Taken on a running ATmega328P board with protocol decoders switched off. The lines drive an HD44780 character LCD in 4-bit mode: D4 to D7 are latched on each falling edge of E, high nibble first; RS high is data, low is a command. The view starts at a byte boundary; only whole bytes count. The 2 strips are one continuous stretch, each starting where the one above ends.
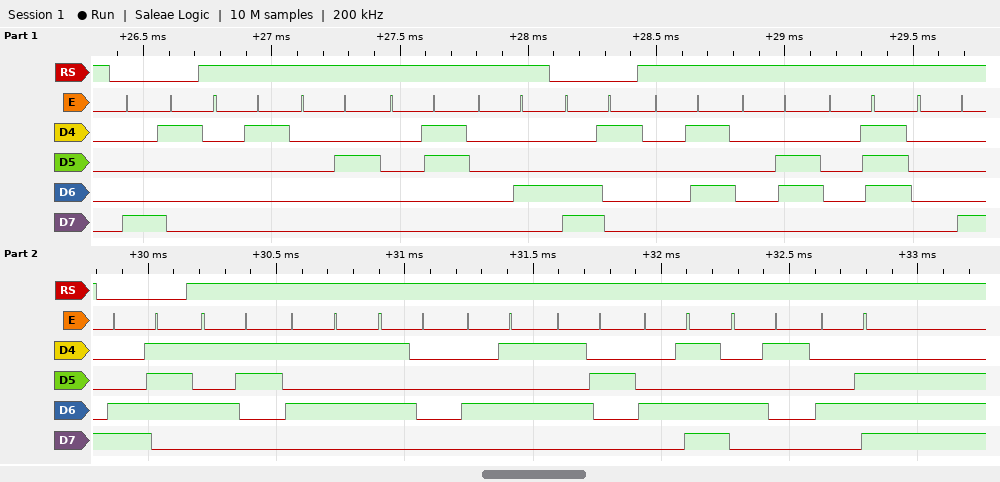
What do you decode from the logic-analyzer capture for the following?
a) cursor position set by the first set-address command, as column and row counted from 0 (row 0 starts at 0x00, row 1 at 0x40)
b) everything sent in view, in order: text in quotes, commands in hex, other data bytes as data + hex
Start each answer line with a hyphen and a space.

- column 1, row 0
- 0x81 data 01 02 03 04 0xC1 data 05 06 07 08 0xC7 "SUPERMAN"
